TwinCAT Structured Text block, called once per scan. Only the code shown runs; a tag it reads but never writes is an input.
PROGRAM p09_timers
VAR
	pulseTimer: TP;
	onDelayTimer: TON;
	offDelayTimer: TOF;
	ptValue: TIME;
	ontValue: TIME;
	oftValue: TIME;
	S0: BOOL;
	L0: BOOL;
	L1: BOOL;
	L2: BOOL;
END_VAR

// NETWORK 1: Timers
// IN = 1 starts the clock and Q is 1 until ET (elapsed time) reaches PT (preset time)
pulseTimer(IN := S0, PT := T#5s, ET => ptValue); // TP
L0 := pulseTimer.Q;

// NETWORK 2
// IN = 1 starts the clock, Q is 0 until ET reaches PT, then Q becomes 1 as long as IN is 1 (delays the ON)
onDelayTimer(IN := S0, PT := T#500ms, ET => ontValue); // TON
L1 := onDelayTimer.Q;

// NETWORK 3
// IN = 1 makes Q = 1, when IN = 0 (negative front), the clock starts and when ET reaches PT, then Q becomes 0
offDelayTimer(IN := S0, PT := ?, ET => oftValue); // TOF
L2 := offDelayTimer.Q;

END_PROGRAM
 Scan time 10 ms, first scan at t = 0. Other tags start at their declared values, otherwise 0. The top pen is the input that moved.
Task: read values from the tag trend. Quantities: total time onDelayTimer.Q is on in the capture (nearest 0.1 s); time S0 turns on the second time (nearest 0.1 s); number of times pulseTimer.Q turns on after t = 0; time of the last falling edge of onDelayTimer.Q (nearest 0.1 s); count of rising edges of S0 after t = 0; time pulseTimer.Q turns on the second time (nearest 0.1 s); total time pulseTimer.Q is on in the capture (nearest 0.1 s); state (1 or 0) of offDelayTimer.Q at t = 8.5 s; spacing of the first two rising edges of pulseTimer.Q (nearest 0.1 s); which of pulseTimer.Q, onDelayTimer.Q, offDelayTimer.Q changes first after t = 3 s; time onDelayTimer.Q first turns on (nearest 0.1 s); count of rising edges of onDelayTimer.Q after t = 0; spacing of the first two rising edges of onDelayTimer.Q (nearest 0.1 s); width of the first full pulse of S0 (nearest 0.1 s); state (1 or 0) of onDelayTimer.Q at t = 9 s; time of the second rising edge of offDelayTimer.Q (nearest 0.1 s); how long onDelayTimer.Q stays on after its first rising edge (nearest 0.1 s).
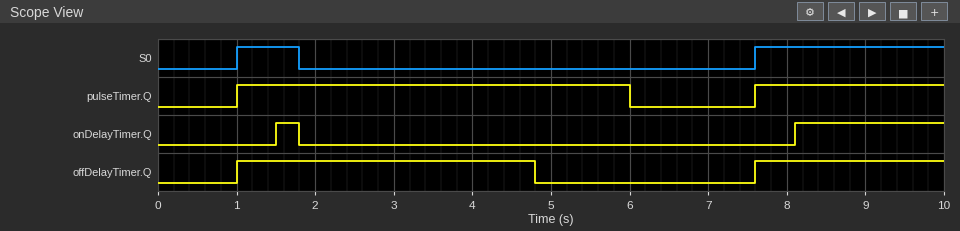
2.2 s
7.6 s
2
1.8 s
2
7.6 s
7.4 s
1
6.6 s
offDelayTimer.Q
1.5 s
2
6.6 s
0.8 s
1
7.6 s
0.3 s
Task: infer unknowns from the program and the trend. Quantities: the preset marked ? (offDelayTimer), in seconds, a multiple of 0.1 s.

3.0 s
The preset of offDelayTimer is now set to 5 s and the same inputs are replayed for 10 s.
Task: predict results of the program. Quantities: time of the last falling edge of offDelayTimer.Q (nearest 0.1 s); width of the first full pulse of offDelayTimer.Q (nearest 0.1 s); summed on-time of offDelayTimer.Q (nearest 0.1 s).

6.8 s
5.8 s
8.2 s
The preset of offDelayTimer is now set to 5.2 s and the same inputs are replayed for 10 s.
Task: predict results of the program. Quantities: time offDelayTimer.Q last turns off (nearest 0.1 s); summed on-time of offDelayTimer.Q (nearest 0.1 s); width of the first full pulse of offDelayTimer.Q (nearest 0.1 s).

7.0 s
8.4 s
6.0 s
